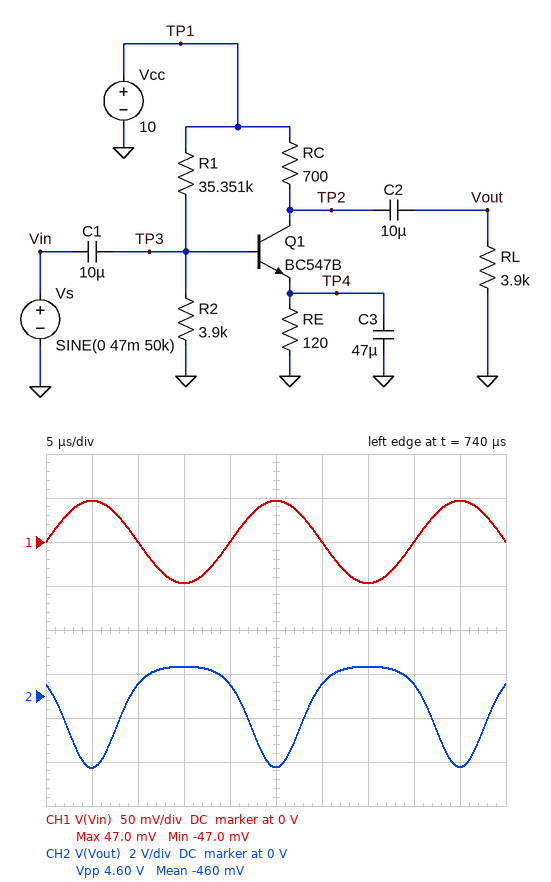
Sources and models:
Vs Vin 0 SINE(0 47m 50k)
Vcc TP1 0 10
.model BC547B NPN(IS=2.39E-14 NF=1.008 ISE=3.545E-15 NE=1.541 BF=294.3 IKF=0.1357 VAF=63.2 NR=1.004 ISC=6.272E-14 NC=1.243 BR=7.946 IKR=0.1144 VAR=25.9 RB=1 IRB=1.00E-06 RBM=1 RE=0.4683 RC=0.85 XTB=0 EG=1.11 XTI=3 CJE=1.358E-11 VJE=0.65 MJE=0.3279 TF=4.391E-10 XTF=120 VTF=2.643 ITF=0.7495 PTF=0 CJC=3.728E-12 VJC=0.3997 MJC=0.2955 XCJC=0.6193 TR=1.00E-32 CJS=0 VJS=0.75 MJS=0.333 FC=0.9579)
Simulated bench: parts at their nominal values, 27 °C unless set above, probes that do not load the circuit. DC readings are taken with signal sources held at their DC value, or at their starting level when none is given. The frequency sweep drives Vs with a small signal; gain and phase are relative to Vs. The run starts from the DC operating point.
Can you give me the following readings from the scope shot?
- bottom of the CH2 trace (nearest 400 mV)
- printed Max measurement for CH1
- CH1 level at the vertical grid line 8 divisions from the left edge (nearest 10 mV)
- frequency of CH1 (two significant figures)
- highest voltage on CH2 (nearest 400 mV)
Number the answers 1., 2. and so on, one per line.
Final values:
1. -3.2 V
2. 47.0 mV
3. 0 V
4. 50 kHz
5. 1.2 V
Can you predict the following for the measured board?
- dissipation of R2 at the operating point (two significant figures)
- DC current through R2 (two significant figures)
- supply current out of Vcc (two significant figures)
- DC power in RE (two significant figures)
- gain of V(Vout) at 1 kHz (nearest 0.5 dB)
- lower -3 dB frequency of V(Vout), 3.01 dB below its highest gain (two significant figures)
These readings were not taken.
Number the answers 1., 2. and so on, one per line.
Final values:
1. 240 µW
2. 250 µA
3. 2.8 mA
4. 770 µW
5. 34.0 dB
6. 330 Hz
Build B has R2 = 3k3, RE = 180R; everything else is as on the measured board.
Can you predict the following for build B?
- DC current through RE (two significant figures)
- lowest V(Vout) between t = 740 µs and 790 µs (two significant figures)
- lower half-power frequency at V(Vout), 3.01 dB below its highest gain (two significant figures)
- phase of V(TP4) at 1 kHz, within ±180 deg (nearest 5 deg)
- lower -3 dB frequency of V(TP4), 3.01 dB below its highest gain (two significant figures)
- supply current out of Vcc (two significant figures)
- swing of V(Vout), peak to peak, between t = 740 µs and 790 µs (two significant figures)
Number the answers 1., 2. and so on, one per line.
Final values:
1. 1.1 mA
2. -1.9 V
3. 160 Hz
4. -80 deg
5. 5.1 Hz
6. 1.4 mA
7. 2.5 V
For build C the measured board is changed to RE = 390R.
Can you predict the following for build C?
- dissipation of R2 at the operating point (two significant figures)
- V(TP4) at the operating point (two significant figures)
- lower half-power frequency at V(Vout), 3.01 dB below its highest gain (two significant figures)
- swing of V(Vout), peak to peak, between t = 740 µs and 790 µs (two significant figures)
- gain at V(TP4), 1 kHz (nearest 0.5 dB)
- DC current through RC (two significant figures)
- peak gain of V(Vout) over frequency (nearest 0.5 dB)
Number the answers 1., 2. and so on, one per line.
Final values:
1. 250 µW
2. 350 mV
3. 120 Hz
4. 2.1 V
5. -19.0 dB
6. 900 µA
7. 26.0 dB
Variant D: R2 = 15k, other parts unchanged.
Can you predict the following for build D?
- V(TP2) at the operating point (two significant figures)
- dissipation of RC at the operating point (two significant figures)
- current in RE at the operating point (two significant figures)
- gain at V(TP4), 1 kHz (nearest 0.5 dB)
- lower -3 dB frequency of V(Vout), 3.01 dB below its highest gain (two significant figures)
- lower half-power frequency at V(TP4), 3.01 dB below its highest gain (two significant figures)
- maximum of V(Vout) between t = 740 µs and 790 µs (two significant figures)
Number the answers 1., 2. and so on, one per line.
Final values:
1. 1.6 V
2. 100 mW
3. 12 mA
4. -12.0 dB
5. 1.1 kHz
6. 22 Hz
7. 6.0 V
